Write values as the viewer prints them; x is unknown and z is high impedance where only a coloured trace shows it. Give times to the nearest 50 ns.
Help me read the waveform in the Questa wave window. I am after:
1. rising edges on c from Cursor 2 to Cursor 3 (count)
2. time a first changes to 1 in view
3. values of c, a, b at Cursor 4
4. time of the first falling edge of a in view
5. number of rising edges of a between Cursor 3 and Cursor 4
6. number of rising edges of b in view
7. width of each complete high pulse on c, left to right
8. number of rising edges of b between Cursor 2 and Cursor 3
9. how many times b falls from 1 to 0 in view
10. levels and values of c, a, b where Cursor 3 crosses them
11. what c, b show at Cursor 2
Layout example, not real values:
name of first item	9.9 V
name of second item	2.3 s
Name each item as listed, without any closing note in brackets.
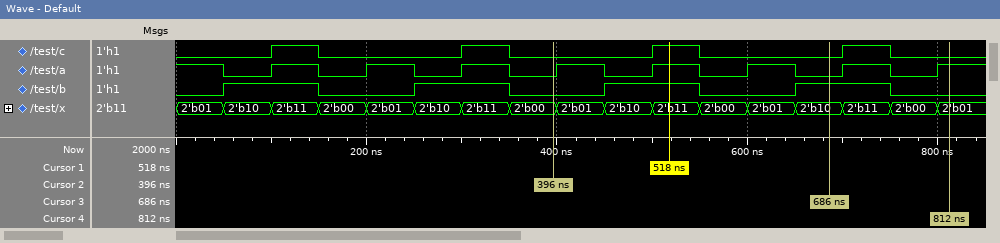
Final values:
rising edges on c from Cursor 2 to Cursor 3	1
time a first changes to 1 in view	100 ns
values of c, a, b at Cursor 4	c=0, a=1, b=0
time of the first falling edge of a in view	50 ns
number of rising edges of a between Cursor 3 and Cursor 4	2
number of rising edges of b in view	4
width of each complete high pulse on c, left to right	50 ns, 50 ns, 50 ns, 50 ns
number of rising edges of b between Cursor 2 and Cursor 3	2
how many times b falls from 1 to 0 in view	4
levels and values of c, a, b where Cursor 3 crosses them	c=0, a=0, b=1
what c, b show at Cursor 2	c=0, b=0
